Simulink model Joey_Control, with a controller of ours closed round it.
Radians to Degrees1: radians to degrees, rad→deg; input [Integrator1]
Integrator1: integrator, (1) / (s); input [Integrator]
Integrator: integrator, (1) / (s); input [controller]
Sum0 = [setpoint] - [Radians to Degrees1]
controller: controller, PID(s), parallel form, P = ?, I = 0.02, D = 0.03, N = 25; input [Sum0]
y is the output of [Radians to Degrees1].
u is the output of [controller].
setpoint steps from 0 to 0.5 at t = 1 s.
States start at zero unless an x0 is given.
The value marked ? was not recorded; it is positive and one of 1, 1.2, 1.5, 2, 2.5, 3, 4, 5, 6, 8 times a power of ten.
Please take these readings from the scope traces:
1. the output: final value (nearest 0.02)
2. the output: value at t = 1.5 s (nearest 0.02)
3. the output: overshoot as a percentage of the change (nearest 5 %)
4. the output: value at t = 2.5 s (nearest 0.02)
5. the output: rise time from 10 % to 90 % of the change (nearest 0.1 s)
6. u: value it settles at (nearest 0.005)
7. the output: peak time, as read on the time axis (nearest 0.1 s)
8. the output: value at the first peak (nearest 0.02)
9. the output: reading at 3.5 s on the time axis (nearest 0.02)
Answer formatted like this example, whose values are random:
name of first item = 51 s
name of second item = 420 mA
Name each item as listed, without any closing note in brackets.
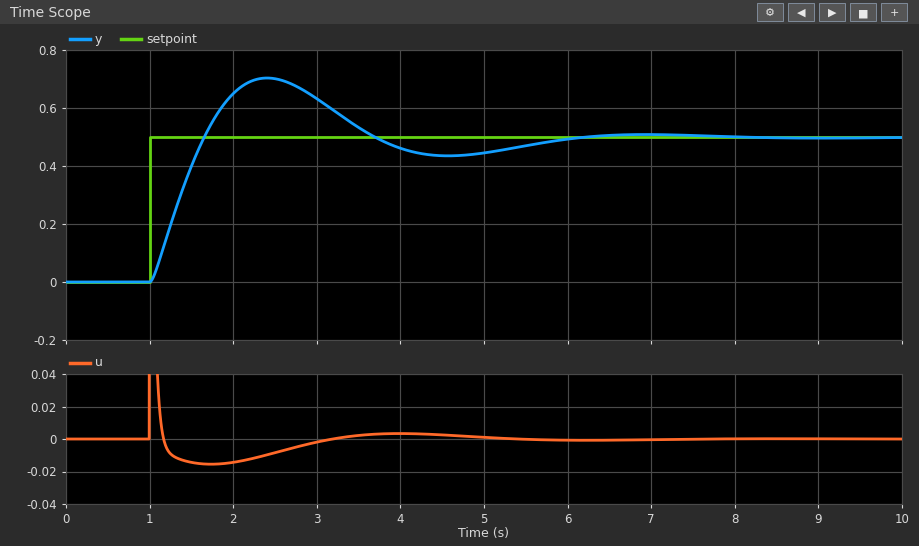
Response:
the output: final value = 0.50
the output: value at t = 1.5 s = 0.40
the output: overshoot as a percentage of the change = 40 %
the output: value at t = 2.5 s = 0.70
the output: rise time from 10 % to 90 % of the change = 0.5 s
u: value it settles at = 0.000
the output: peak time, as read on the time axis = 2.4 s
the output: value at the first peak = 0.70
the output: reading at 3.5 s on the time axis = 0.54
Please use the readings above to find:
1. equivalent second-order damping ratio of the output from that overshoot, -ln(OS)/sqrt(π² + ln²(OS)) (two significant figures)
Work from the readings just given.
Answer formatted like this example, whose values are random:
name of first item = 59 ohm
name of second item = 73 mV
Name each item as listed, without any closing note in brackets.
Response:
equivalent second-order damping ratio of the output from that overshoot, -ln(OS)/sqrt(π² + ln²(OS)) = 0.28
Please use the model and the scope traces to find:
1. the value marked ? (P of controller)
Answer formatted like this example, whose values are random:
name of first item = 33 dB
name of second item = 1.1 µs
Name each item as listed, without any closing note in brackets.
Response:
the value marked ? = 0.05
